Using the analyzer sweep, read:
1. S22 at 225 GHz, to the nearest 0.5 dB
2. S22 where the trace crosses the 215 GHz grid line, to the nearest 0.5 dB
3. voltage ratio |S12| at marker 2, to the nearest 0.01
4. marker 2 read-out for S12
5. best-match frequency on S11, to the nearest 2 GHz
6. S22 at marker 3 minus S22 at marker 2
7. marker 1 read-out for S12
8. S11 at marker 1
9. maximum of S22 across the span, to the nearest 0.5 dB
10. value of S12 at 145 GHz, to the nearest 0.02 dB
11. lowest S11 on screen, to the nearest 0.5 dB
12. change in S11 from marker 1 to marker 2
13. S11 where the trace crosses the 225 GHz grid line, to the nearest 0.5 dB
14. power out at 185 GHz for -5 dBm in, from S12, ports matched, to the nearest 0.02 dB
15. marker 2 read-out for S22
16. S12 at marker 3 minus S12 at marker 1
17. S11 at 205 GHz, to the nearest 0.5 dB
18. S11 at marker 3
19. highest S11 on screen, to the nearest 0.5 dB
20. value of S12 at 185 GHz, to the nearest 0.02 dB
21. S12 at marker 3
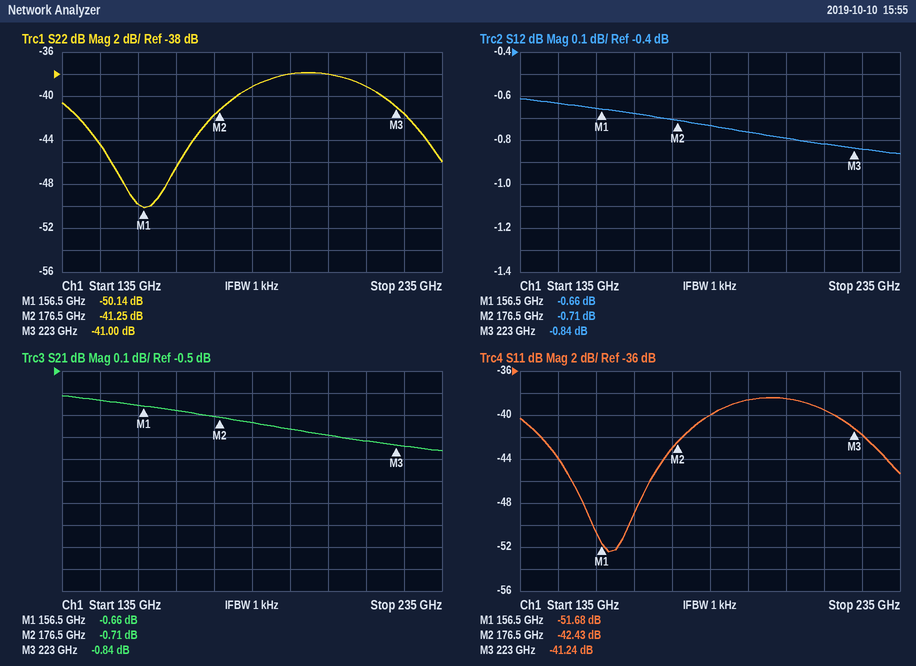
-41.5 dB
-39.0 dB
0.92
-0.71 dB
158 GHz
0.25 dB
-0.66 dB
-51.68 dB
-38.0 dB
-0.64 dB
-52.5 dB
9.25 dB
-42.0 dB
-5.74 dBm
-41.25 dB
-0.18 dB
-38.5 dB
-41.24 dB
-38.5 dB
-0.74 dB
-0.84 dB
